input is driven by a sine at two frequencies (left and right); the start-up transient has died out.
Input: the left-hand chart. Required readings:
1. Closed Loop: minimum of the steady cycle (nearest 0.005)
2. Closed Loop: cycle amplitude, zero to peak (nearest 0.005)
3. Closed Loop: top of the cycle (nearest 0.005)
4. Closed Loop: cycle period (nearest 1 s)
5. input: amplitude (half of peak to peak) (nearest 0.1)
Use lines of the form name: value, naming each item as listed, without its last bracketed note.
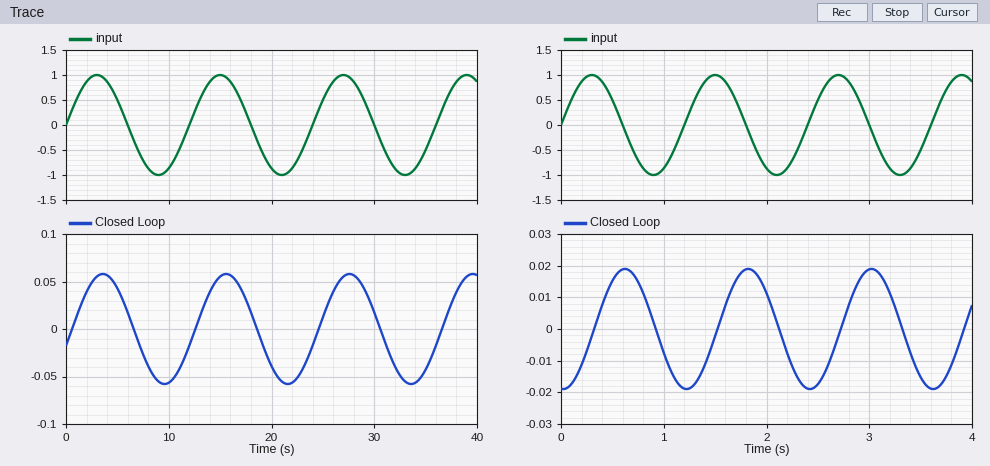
Closed Loop: minimum of the steady cycle: -0.060
Closed Loop: cycle amplitude, zero to peak: 0.060
Closed Loop: top of the cycle: 0.060
Closed Loop: cycle period: 12 s
input: amplitude (half of peak to peak): 1.0
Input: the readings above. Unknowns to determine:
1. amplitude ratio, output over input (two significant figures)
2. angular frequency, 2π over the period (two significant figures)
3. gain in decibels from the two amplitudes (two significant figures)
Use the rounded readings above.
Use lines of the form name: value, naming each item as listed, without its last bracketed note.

amplitude ratio, output over input: 0.060
angular frequency, 2π over the period: 0.52 rad/s
gain in decibels from the two amplitudes: -24 dB
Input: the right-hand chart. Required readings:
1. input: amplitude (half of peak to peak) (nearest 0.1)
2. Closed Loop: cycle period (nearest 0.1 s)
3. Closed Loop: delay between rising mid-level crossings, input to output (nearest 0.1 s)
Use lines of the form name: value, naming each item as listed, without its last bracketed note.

input: amplitude (half of peak to peak): 1.0
Closed Loop: cycle period: 1.2 s
Closed Loop: delay between rising mid-level crossings, input to output: 0.3 s
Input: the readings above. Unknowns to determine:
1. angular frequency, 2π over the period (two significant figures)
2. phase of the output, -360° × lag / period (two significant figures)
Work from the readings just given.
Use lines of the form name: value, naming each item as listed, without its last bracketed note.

angular frequency, 2π over the period: 5.2 rad/s
phase of the output, -360° × lag / period: -90°
